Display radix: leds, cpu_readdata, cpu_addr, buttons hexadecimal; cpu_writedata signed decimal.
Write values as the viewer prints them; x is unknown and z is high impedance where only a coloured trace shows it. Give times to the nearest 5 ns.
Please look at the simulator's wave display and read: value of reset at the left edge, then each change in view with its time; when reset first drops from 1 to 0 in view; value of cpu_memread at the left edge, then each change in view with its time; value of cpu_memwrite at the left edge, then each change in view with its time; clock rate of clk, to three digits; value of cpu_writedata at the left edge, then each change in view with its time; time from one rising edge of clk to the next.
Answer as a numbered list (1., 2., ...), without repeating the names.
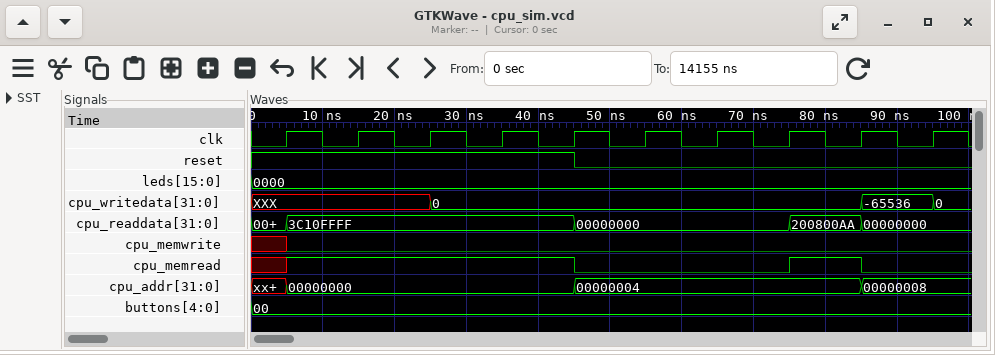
1. 1, 0 at 45 ns
2. 45 ns
3. x, 1 at 5 ns, 0 at 45 ns, 1 at 75 ns, 0 at 85 ns
4. x, 0 at 5 ns
5. 100 MHz
6. XXX, 0 at 25 ns, -65536 at 85 ns, 0 at 95 ns
7. 10 ns
